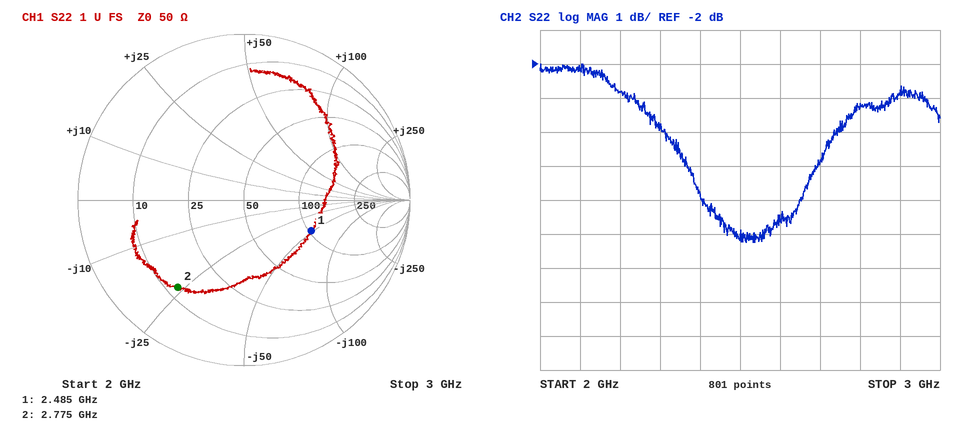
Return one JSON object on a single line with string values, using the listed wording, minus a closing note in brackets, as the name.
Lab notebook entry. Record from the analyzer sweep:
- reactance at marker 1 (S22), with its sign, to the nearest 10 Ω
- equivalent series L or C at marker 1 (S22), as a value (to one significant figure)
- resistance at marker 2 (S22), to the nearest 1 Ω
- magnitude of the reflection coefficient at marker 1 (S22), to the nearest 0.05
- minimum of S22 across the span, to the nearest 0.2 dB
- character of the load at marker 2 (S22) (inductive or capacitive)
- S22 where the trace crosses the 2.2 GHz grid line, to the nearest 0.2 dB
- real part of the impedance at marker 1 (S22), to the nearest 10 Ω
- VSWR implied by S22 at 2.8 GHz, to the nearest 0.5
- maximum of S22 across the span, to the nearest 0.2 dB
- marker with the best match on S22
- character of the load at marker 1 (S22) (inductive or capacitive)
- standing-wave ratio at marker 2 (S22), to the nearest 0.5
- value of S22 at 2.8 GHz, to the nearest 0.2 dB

{"reactance at marker 1 (S22), with its sign, to the nearest 10 Ω": "-50 Ω", "equivalent series L or C at marker 1 (S22), as a value": "1 pF", "resistance at marker 2 (S22), to the nearest 1 Ω": "13 Ω", "magnitude of the reflection coefficient at marker 1 (S22), to the nearest 0.05": "0.45", "minimum of S22 across the span, to the nearest 0.2 dB": "-7.2 dB", "character of the load at marker 2 (S22)": "capacitive", "S22 where the trace crosses the 2.2 GHz grid line, to the nearest 0.2 dB": "-2.8 dB", "real part of the impedance at marker 1 (S22), to the nearest 10 Ω": "100 Ω", "VSWR implied by S22 at 2.8 GHz, to the nearest 0.5": "5.5", "maximum of S22 across the span, to the nearest 0.2 dB": "-2.0 dB", "marker with the best match on S22": "marker 1", "character of the load at marker 1 (S22)": "capacitive", "standing-wave ratio at marker 2 (S22), to the nearest 0.5": "5.0", "value of S22 at 2.8 GHz, to the nearest 0.2 dB": "-3.2 dB"}
